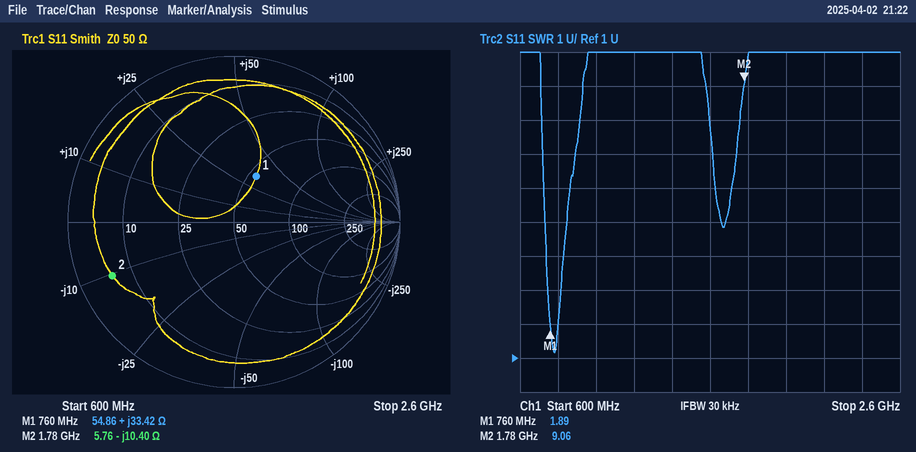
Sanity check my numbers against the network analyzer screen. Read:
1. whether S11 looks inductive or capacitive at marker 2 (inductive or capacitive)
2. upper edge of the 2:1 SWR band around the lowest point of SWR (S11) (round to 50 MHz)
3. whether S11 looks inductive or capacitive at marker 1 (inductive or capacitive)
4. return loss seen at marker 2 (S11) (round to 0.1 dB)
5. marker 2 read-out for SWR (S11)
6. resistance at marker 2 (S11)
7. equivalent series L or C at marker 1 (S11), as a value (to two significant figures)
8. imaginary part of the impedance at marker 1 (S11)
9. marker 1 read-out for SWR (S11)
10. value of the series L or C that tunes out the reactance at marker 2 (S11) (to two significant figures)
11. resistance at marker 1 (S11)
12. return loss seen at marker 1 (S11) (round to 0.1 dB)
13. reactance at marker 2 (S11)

capacitive
800 MHz
inductive
1.9 dB
9.06
5.76 Ω
7.0 nH
+33.42 Ω
1.89
930 pH
54.86 Ω
10.3 dB
-10.40 Ω
